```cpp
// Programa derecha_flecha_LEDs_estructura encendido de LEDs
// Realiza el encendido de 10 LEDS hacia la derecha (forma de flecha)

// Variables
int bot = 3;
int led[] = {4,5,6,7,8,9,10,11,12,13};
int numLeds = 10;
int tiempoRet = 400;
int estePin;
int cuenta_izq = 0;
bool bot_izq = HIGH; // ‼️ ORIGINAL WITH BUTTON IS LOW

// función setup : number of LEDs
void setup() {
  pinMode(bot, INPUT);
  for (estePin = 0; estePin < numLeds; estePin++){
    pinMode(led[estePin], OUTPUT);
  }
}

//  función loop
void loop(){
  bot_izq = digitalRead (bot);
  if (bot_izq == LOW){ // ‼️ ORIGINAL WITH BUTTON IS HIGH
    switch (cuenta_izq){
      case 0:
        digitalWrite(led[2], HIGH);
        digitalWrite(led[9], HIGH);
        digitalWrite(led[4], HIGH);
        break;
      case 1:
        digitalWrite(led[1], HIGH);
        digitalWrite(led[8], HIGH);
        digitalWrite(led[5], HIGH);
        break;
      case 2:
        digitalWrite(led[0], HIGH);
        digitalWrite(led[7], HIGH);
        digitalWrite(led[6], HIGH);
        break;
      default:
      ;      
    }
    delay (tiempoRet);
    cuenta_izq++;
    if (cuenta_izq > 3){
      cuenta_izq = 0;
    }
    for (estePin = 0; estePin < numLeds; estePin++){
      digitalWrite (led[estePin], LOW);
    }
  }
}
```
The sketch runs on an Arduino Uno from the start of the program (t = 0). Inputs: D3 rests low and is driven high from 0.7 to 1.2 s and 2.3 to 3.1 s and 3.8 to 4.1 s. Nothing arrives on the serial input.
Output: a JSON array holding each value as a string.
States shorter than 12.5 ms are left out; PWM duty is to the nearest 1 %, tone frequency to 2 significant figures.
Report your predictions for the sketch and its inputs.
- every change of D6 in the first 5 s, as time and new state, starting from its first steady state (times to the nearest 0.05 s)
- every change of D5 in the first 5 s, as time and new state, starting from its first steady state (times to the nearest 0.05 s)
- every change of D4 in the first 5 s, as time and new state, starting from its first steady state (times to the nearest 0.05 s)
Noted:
["0 s high; 0.4 s low; 2 s high; 2.4 s low; 4.5 s high; 4.9 s low", "0 s low; 0.4 s high; 0.8 s low; 3.1 s high; 3.5 s low; 4.9 s high", "0 s low; 1.2 s high; 1.6 s low; 3.5 s high; 3.9 s low"]
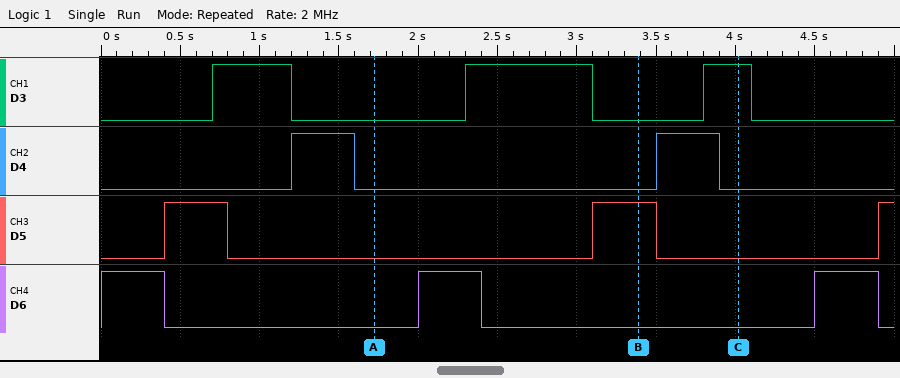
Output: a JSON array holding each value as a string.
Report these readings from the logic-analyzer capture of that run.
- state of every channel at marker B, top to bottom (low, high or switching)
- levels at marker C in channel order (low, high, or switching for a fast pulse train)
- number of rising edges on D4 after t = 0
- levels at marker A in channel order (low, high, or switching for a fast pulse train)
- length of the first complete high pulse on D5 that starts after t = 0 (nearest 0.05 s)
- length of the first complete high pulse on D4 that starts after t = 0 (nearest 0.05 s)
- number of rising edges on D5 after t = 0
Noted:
["D3 low, D4 low, D5 high, D6 low", "D3 high, D4 low, D5 low, D6 low", "2", "D3 low, D4 low, D5 low, D6 low", "0.40 s", "0.40 s", "3"]
